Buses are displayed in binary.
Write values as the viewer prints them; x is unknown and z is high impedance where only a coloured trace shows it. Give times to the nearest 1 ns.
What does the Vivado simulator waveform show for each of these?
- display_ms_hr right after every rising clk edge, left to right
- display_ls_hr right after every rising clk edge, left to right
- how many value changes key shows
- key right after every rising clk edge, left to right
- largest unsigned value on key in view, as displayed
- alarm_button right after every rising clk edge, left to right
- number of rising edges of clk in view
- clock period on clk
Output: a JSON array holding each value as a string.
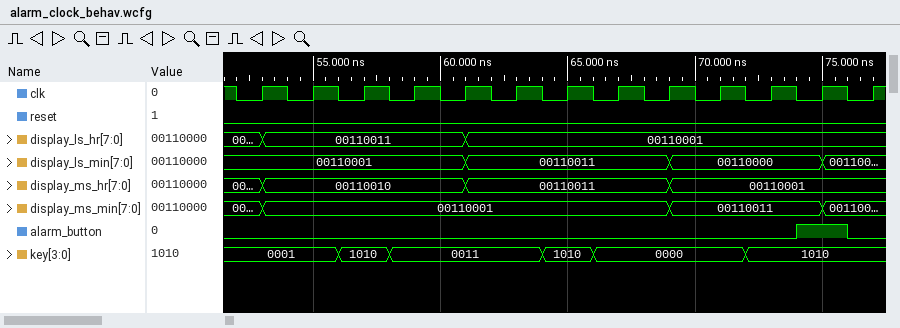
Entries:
["00110010, 00110010, 00110010, 00110010, 00110011, 00110011, 00110011, 00110011, 00110001, 00110001, 00110001, 00110001, 00110001", "00110011, 00110011, 00110011, 00110011, 00110001, 00110001, 00110001, 00110001, 00110001, 00110001, 00110001, 00110001, 00110001", "5", "0001, 0001, 1010, 0011, 0011, 0011, 1010, 0000, 0000, 0000, 1010, 1010, 1010", "1010", "0 0 0 0 0 0 0 0 0 0 0 1 0", "13", "2 ns"]
